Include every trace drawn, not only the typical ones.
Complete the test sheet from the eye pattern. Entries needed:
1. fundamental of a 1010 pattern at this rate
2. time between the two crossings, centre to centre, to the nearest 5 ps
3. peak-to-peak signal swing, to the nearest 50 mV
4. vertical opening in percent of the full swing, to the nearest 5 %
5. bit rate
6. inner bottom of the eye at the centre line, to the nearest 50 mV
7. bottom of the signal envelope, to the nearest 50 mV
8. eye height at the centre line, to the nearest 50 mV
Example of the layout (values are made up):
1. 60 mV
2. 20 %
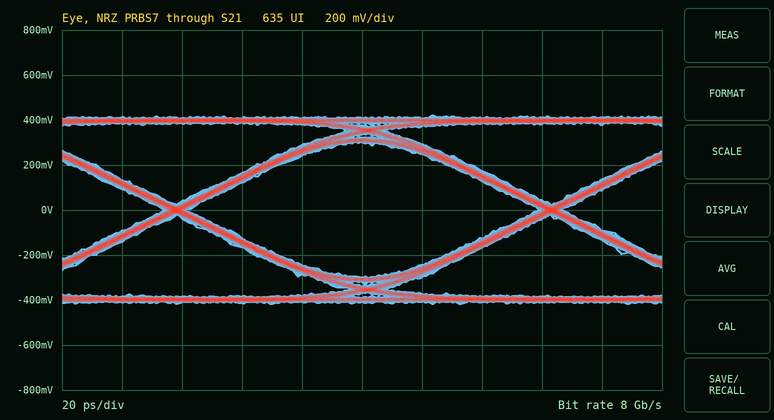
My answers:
1. 4 GHz
2. 125 ps
3. 850 mV
4. 70 %
5. 8 Gb/s
6. -300 mV
7. -400 mV
8. 600 mV
